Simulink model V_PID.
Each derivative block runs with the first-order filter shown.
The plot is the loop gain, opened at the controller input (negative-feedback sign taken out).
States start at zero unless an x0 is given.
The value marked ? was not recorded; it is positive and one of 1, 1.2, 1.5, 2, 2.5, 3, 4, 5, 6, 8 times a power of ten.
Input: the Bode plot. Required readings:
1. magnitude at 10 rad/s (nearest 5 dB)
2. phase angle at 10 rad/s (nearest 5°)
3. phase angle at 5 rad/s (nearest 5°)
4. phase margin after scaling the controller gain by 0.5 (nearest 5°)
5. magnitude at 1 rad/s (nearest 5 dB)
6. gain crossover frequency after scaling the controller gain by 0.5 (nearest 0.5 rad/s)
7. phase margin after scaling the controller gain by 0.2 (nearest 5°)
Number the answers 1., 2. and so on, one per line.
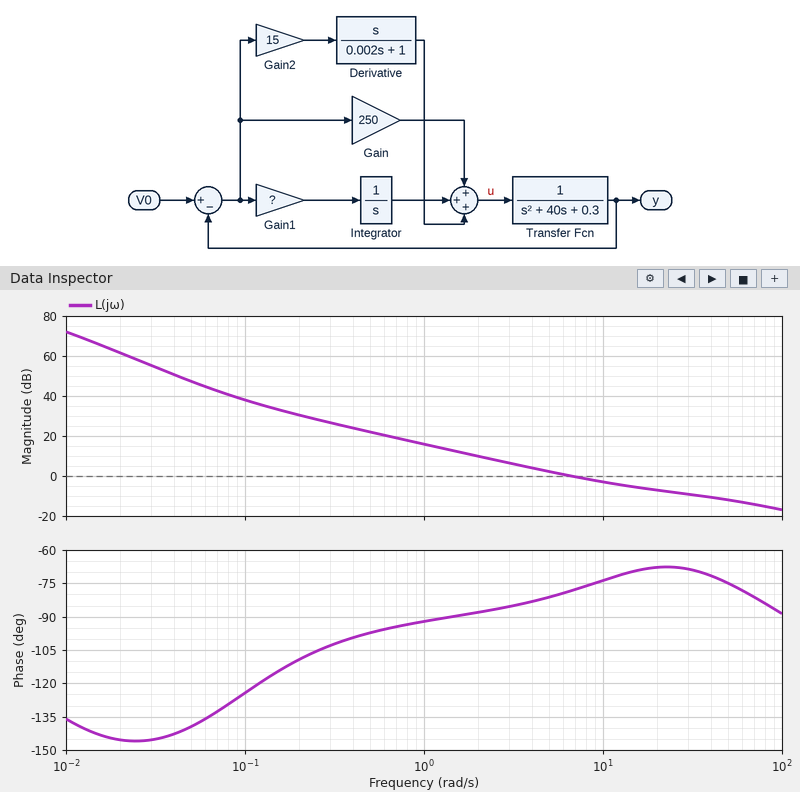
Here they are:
1. -5 dB
2. -75°
3. -80°
4. 95°
5. 15 dB
6. 3.0 rad/s
7. 90°
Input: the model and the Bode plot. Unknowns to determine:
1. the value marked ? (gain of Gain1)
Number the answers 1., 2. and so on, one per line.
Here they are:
1. 20
